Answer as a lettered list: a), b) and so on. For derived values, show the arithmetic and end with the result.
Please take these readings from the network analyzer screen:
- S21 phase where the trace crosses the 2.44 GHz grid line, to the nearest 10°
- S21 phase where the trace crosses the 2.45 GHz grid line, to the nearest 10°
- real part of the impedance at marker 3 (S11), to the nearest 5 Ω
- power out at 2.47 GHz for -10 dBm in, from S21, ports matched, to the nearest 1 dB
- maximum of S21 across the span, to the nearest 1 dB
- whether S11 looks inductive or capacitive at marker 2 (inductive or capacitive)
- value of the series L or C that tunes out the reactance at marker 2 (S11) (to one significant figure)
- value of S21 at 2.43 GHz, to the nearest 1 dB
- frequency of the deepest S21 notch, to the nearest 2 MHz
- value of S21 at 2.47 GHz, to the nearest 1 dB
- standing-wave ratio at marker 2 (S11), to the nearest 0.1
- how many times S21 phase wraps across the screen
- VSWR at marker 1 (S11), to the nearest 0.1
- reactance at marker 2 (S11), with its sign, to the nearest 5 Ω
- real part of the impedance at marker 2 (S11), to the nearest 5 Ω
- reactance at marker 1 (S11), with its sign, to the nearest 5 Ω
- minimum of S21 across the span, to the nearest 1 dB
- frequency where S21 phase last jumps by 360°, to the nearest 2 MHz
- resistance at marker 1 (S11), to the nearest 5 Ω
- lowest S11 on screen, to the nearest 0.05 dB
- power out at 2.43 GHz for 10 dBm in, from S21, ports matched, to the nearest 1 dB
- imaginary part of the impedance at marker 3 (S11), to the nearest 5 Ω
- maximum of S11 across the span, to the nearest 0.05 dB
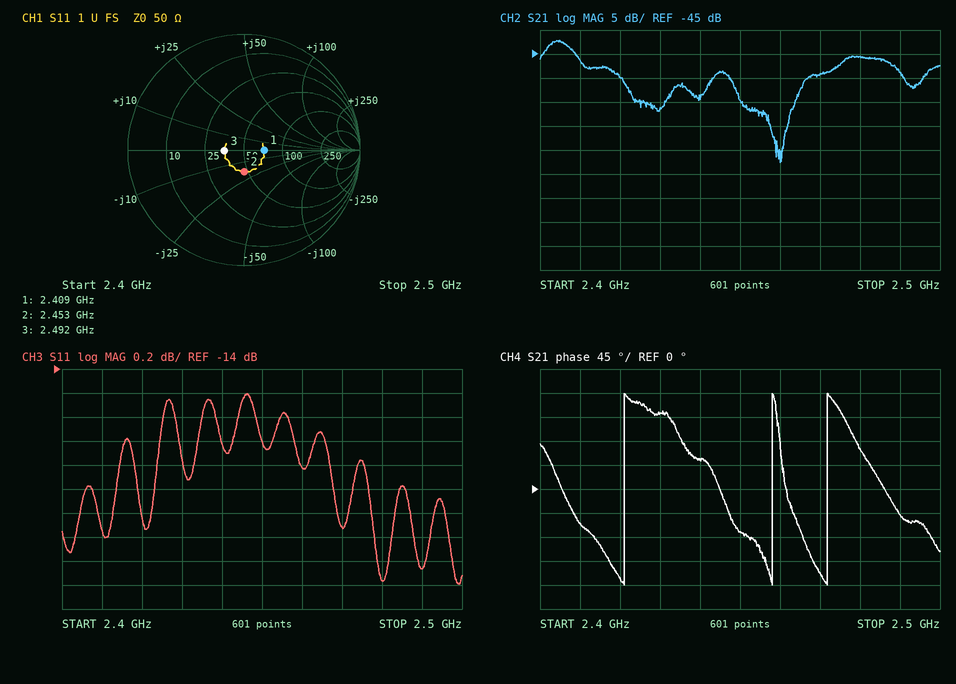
a) 60°
b) -80°
c) 35 Ω
d) -10 dBm + (-49 dB) = -59 dBm
e) -42 dB
f) capacitive
g) L = 20 Ω/(2π × 2.453 GHz) ≈ 1 nH
h) -56 dB
i) 2.460 GHz
j) -49 dB
k) 1.5
l) 3
m) 1.4
n) -20 Ω
o) 45 Ω
p) 0 Ω
q) -68 dB
r) 2.472 GHz
s) 70 Ω
t) -15.80 dB
u) 10 dBm + (-56 dB) = -46 dBm
v) 0 Ω
w) -14.20 dB
